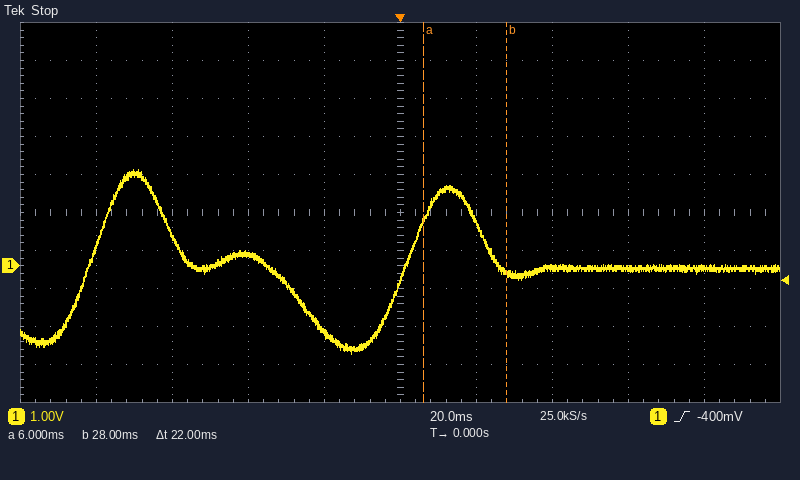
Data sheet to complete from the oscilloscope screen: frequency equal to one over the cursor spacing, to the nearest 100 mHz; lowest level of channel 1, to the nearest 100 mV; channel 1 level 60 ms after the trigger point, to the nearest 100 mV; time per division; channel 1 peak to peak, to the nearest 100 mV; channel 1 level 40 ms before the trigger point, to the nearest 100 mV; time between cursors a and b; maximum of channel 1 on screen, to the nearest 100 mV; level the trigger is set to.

45.5 Hz
-2.3 V
-100 mV
20 ms
4.8 V
300 mV
22 ms
2.5 V
-400 mV
